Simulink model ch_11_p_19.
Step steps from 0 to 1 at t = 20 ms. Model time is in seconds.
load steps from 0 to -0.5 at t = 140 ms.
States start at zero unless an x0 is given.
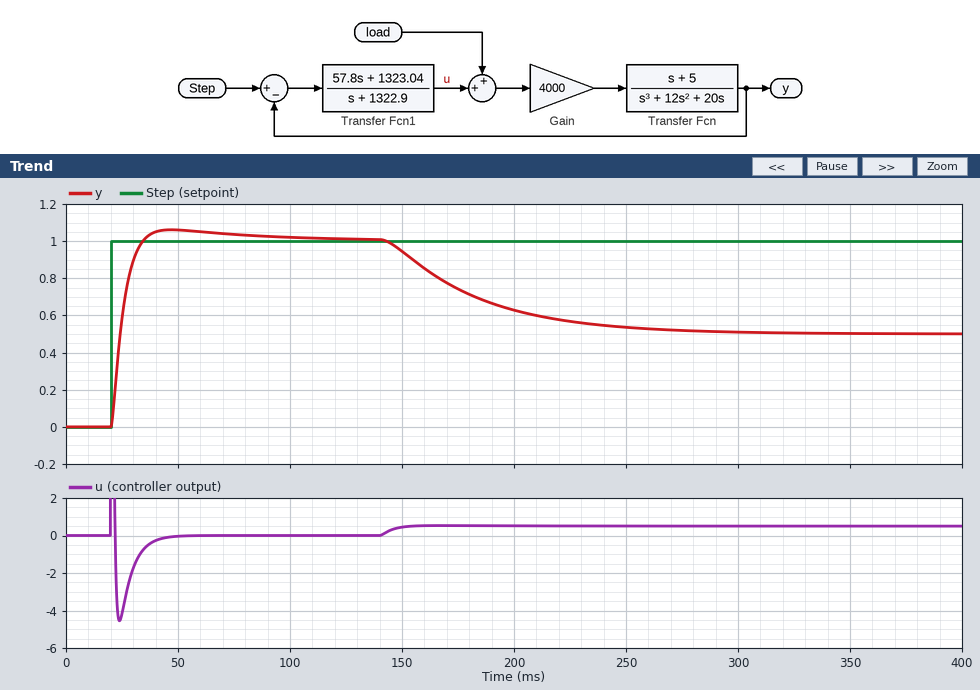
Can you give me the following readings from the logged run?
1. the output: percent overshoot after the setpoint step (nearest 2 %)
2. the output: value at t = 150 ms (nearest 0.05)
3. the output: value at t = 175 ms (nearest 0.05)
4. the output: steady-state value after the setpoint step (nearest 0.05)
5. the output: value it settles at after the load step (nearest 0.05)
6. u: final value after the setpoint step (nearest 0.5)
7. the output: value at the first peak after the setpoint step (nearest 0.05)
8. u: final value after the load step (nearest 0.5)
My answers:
6 %
0.95
0.75
1.00
0.50
0.0
1.05
0.5
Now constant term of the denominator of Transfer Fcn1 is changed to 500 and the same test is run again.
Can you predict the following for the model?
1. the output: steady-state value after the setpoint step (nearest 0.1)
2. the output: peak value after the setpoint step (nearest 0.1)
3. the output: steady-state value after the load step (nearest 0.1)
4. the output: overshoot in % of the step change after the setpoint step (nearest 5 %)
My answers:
1.0
1.2
0.8
20 %
